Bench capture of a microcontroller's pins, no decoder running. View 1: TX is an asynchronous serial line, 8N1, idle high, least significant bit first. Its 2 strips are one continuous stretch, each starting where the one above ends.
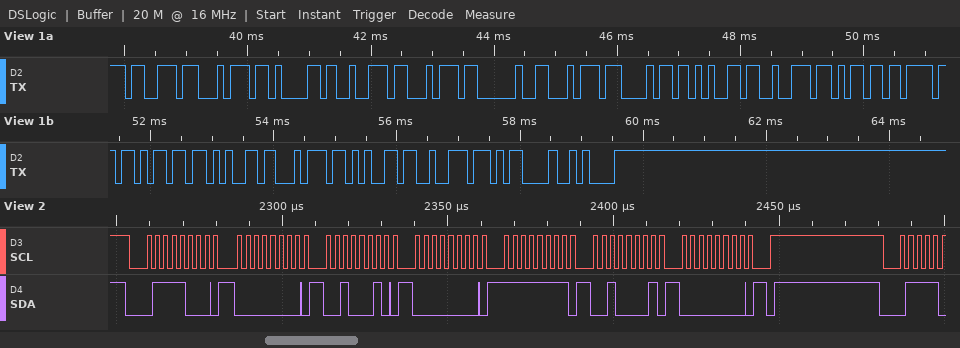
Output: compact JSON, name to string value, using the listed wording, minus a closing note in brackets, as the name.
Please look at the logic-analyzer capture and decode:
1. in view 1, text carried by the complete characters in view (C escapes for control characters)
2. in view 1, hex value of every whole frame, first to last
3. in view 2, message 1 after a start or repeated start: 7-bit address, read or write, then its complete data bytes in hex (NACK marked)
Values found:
{"in view 1, text carried by the complete characters in view": "\"start thermometer\\r\\n\"", "in view 1, hex value of every whole frame, first to last": "0x73 0x74 0x61 0x72 0x74 0x20 0x74 0x68 0x65 0x72 0x6D 0x6F 0x6D 0x65 0x74 0x65 0x72 0x0D 0x0A", "in view 2, message 1 after a start or repeated start: 7-bit address, read or write, then its complete data bytes in hex": "0x3C write: 00 22 00 FF 21 00"}
